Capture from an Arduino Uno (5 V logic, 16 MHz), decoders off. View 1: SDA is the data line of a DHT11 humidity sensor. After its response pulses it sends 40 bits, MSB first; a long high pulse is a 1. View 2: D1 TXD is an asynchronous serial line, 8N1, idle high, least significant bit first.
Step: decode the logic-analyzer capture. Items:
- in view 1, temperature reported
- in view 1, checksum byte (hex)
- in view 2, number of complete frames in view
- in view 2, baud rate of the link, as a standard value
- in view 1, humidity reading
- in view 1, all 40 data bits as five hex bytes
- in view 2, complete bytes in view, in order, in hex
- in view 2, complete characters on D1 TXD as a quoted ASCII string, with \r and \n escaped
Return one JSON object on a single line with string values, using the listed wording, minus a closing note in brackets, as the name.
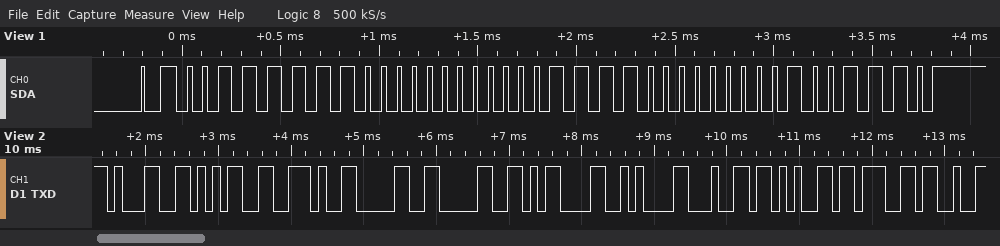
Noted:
{"in view 1, temperature reported": "15.0 °C", "in view 1, checksum byte": "0x4E", "in view 2, number of complete frames in view": "10", "in view 2, baud rate of the link, as a standard value": "9600 baud", "in view 1, humidity reading": "63 %", "in view 1, all 40 data bits as five hex bytes": "3F 00 0F 00 4E", "in view 2, complete bytes in view, in order, in hex": "0x31 0x35 0x2E 0x30 0x30 0x0D 0x0A 0x64 0x65 0x67", "in view 2, complete characters on D1 TXD as a quoted ASCII string, with \\r and \\n escaped": "\"15.00\\r\\ndeg\""}
